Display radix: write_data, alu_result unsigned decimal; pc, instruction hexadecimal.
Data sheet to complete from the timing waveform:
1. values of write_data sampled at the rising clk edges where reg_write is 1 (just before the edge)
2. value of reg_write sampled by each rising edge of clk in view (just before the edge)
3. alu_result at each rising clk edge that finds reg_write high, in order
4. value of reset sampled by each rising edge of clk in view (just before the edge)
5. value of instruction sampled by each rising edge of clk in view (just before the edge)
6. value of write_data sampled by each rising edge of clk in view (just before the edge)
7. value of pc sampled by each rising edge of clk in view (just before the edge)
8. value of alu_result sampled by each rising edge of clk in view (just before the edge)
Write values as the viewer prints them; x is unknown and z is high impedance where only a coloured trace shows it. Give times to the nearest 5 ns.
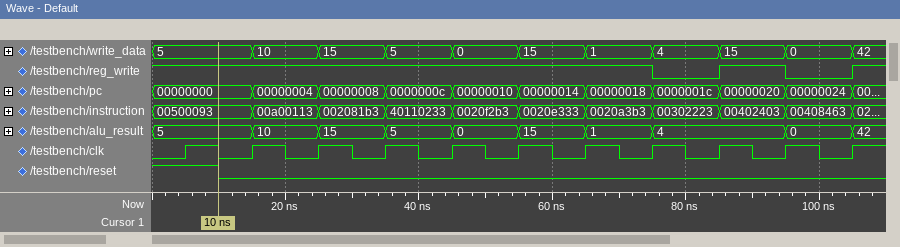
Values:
5, 5, 10, 15, 5, 0, 15, 1, 15
1 1 1 1 1 1 1 1 0 1 0
5, 5, 10, 15, 5, 0, 15, 1, 4
1 0 0 0 0 0 0 0 0 0 0
00500093, 00500093, 00a00113, 002081b3, 40110233, 0020f2b3, 0020e333, 0020a3b3, 00302223, 00402403, 00408463
5, 5, 10, 15, 5, 0, 15, 1, 4, 15, 0
00000000, 00000000, 00000004, 00000008, 0000000c, 00000010, 00000014, 00000018, 0000001c, 00000020, 00000024
5, 5, 10, 15, 5, 0, 15, 1, 4, 4, 0
